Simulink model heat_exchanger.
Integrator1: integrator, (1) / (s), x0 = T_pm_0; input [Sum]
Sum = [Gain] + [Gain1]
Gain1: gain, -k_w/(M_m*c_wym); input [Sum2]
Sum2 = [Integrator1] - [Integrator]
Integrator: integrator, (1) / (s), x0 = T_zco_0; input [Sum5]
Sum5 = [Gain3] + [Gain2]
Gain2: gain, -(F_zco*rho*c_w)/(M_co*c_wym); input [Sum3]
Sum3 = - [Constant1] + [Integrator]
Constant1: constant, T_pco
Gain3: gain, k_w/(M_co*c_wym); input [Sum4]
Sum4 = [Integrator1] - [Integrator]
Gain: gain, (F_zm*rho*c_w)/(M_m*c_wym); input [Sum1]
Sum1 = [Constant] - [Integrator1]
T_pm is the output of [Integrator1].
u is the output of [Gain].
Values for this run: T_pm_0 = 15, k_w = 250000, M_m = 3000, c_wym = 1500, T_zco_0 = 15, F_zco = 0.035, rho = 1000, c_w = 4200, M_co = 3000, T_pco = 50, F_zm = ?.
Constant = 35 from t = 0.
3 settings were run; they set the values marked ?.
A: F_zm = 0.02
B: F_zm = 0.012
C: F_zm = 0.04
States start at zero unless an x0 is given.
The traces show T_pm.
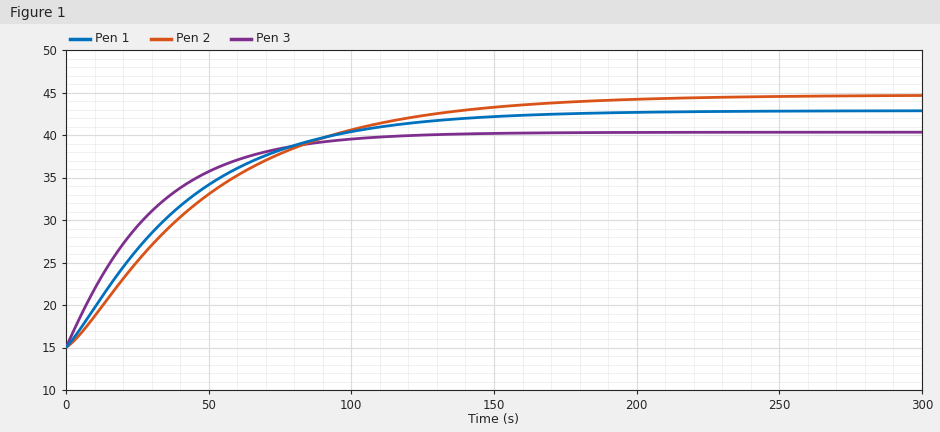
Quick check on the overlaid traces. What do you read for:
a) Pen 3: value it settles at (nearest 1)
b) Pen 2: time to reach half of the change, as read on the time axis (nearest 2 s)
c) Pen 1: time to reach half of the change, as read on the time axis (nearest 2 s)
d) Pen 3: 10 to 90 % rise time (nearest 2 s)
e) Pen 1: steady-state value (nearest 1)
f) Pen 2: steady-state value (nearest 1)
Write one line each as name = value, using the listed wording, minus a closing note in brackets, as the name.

Pen 3: value it settles at = 40
Pen 2: time to reach half of the change, as read on the time axis = 38 s
Pen 1: time to reach half of the change, as read on the time axis = 32 s
Pen 3: 10 to 90 % rise time = 64 s
Pen 1: steady-state value = 43
Pen 2: steady-state value = 45
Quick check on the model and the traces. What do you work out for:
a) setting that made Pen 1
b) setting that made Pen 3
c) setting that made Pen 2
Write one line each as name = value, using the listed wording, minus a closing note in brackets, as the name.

setting that made Pen 1 = A
setting that made Pen 3 = C
setting that made Pen 2 = B
